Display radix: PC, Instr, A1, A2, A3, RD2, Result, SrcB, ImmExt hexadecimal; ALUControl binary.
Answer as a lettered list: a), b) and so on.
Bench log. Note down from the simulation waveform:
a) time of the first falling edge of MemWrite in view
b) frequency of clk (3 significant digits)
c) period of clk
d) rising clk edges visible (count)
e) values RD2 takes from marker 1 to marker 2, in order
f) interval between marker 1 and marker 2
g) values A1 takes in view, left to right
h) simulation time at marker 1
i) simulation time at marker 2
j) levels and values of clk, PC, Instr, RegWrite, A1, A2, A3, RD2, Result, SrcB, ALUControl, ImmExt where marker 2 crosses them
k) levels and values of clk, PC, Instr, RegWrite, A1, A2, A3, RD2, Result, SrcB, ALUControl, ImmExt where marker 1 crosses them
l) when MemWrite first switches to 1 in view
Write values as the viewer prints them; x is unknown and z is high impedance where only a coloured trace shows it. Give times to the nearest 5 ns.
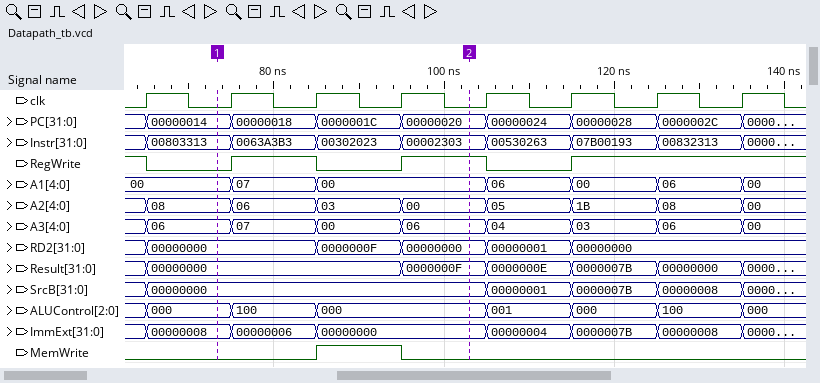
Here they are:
a) 95 ns
b) 100 MHz
c) 10 ns
d) 8
e) 00000000, 0000000F, 00000000
f) 30 ns
g) 00, 07, 00, 06, 00, 06, 00
h) 75 ns
i) 105 ns
j) clk=0, PC=00000020, Instr=00002303, RegWrite=1, A1=00, A2=00, A3=06, RD2=00000000, Result=0000000F, SrcB=00000000, ALUControl=000, ImmExt=00000000
k) clk=0, PC=00000014, Instr=00803313, RegWrite=0, A1=00, A2=08, A3=06, RD2=00000000, Result=00000000, SrcB=00000000, ALUControl=000, ImmExt=00000008
l) 85 ns
